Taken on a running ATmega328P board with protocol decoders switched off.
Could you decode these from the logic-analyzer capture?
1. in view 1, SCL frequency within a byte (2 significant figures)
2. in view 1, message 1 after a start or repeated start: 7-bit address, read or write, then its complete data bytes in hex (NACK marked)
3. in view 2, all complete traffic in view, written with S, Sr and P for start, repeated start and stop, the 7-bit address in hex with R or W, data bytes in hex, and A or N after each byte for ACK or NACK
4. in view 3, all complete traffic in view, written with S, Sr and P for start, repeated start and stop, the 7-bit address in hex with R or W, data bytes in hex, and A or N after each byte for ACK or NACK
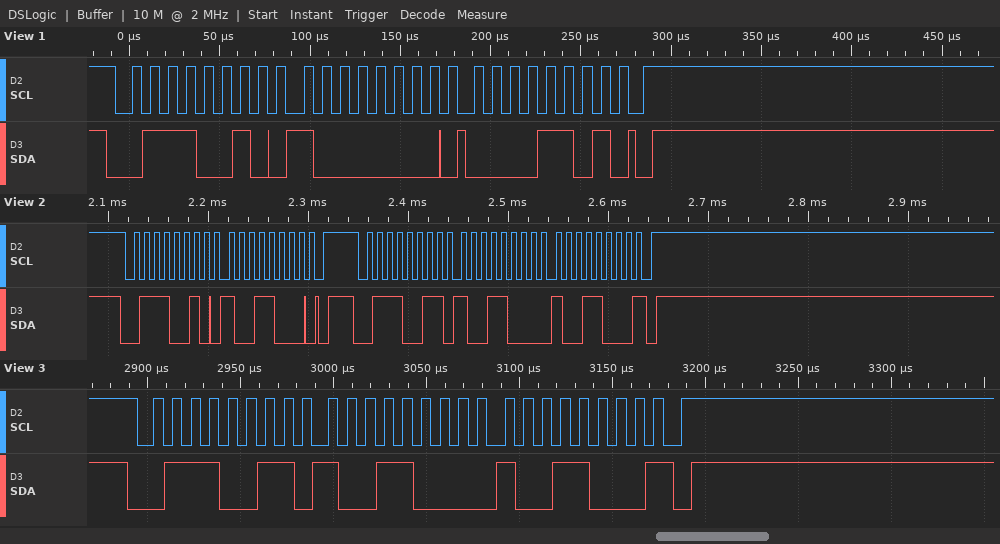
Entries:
100 kHz
0x39 write: 80 0D
S 39W A 98 A P S 39R A 98 A 98 N P
S 39R A 98 A 98 N P
